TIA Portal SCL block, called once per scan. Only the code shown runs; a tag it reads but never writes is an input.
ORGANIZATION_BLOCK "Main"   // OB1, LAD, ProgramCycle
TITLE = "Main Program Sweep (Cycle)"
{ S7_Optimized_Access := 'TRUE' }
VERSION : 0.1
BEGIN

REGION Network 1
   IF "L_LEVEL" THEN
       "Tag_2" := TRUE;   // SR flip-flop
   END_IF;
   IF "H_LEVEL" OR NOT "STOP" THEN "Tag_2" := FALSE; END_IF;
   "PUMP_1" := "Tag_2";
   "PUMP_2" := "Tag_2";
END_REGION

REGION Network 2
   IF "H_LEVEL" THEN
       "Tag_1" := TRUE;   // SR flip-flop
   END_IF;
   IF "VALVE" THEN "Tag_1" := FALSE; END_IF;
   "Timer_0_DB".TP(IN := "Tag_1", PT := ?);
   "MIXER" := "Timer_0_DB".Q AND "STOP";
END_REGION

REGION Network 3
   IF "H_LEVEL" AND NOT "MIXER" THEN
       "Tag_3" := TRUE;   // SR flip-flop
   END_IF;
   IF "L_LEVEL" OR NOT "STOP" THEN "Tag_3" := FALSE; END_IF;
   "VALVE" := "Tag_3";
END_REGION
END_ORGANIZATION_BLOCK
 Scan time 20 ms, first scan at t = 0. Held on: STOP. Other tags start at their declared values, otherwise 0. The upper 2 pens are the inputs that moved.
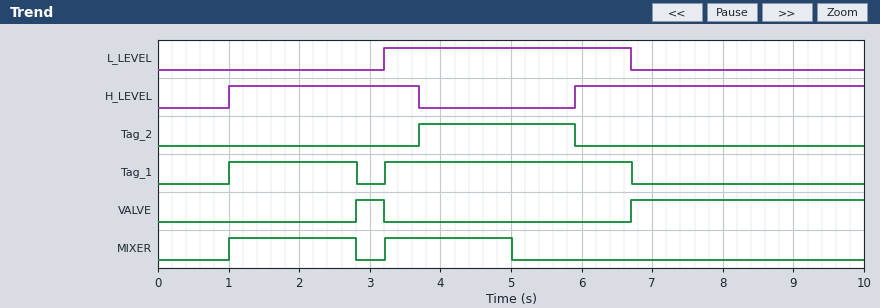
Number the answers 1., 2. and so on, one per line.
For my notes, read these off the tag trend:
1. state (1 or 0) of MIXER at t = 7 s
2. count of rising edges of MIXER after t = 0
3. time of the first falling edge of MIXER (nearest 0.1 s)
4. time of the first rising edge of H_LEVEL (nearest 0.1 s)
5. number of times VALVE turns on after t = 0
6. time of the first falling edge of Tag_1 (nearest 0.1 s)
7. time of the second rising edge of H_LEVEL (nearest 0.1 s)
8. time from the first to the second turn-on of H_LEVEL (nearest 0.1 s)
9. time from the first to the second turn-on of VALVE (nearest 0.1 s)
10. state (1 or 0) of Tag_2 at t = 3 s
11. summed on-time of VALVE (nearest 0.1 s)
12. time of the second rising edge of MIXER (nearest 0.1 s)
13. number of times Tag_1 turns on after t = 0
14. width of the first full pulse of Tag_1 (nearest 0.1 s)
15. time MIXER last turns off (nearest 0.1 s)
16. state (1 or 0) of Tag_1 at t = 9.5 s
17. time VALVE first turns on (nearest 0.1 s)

1. 0
2. 2
3. 2.8 s
4. 1.0 s
5. 2
6. 2.8 s
7. 5.9 s
8. 4.9 s
9. 3.9 s
10. 0
11. 3.7 s
12. 3.2 s
13. 2
14. 1.8 s
15. 5.0 s
16. 0
17. 2.8 s
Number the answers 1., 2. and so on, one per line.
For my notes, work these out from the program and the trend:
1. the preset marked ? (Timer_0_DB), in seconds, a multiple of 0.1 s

1. 1.8 s
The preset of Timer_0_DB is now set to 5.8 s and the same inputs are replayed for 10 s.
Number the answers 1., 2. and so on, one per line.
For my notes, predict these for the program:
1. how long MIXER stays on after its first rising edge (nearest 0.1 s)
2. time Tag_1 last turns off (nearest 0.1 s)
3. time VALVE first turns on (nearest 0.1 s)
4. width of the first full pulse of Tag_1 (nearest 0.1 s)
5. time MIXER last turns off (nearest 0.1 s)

1. 5.8 s
2. 6.8 s
3. 6.8 s
4. 5.8 s
5. 6.8 s
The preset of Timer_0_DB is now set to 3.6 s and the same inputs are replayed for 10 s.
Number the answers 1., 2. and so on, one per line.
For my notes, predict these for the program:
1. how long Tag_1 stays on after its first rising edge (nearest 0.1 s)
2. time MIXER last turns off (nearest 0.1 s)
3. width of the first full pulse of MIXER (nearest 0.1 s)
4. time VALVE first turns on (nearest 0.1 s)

1. 5.7 s
2. 4.6 s
3. 3.6 s
4. 6.7 s
